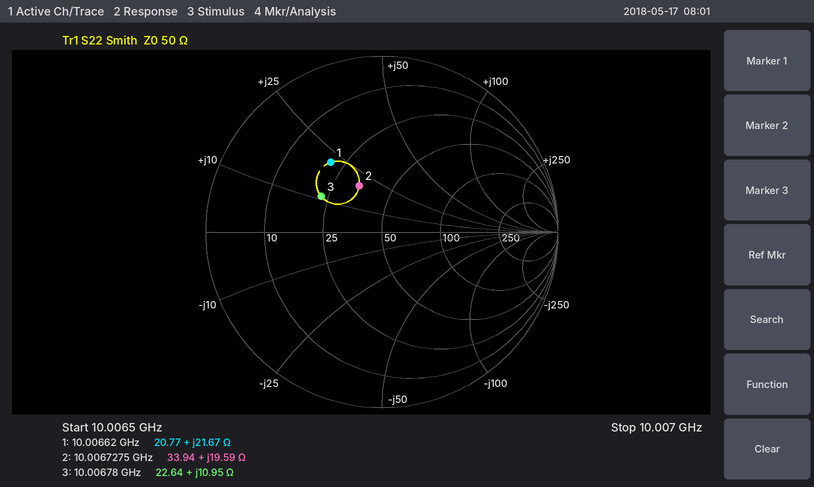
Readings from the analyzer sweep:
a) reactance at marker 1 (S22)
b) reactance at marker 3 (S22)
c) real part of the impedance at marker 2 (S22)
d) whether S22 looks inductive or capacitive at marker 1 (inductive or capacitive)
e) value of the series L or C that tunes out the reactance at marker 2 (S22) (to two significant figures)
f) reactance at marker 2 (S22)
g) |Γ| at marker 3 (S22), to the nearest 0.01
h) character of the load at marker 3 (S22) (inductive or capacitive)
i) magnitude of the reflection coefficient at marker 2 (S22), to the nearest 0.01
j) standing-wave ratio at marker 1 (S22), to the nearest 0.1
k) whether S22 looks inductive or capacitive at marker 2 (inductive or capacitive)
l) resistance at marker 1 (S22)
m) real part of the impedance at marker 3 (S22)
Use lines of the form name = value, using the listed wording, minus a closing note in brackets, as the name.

reactance at marker 1 = +21.67 Ω
reactance at marker 3 = +10.95 Ω
real part of the impedance at marker 2 = 33.94 Ω
whether S22 looks inductive or capacitive at marker 1 = inductive
value of the series L or C that tunes out the reactance at marker 2 (S22) = 810 fF
reactance at marker 2 = +19.59 Ω
|Γ| at marker 3 (S22), to the nearest 0.01 = 0.40
character of the load at marker 3 (S22) = inductive
magnitude of the reflection coefficient at marker 2 (S22), to the nearest 0.01 = 0.29
standing-wave ratio at marker 1 (S22), to the nearest 0.1 = 2.9
whether S22 looks inductive or capacitive at marker 2 = inductive
resistance at marker 1 = 20.77 Ω
real part of the impedance at marker 3 = 22.64 Ω
